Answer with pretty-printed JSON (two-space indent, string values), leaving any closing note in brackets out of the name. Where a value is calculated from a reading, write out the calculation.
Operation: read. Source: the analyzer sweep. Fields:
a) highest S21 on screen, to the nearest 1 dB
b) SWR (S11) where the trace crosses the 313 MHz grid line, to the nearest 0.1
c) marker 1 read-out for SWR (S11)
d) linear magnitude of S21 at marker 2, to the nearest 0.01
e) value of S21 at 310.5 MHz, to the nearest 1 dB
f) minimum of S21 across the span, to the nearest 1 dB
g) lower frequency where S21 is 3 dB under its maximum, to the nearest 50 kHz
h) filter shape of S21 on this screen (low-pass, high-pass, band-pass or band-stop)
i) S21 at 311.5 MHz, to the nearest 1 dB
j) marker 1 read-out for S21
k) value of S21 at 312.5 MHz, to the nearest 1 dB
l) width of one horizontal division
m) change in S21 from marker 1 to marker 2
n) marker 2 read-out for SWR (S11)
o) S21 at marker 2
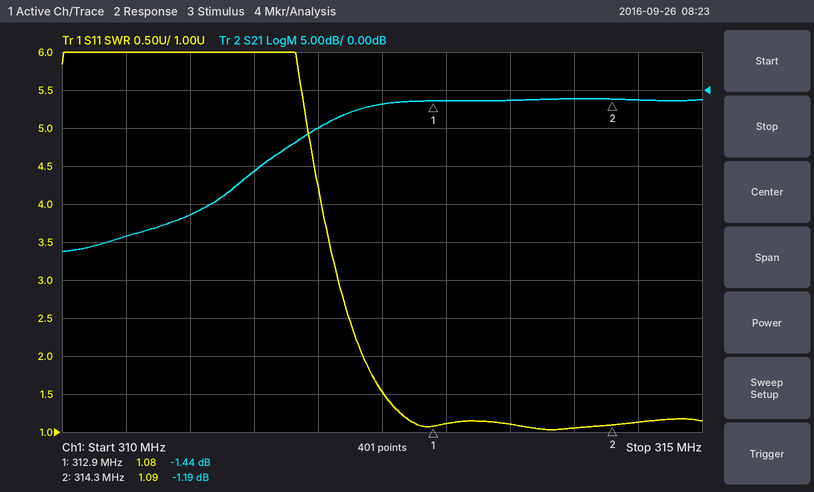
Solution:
{
  "highest S21 on screen, to the nearest 1 dB": "-1 dB",
  "SWR (S11) where the trace crosses the 313 MHz grid line, to the nearest 0.1": "1.1",
  "marker 1 read-out for SWR": "1.08",
  "linear magnitude of S21 at marker 2, to the nearest 0.01": "10^(-1.19/20) ≈ 0.87",
  "value of S21 at 310.5 MHz, to the nearest 1 dB": "-19 dB",
  "minimum of S21 across the span, to the nearest 1 dB": "-21 dB",
  "lower frequency where S21 is 3 dB under its maximum, to the nearest 50 kHz": "312.10 MHz",
  "filter shape of S21 on this screen": "high-pass",
  "S21 at 311.5 MHz, to the nearest 1 dB": "-11 dB",
  "marker 1 read-out for S21": "-1.44 dB",
  "value of S21 at 312.5 MHz, to the nearest 1 dB": "-2 dB",
  "width of one horizontal division": "500 kHz",
  "change in S21 from marker 1 to marker 2": "-1.19 − (-1.44) = 0.25 dB",
  "marker 2 read-out for SWR": "1.09",
  "S21 at marker 2": "-1.19 dB"
}
